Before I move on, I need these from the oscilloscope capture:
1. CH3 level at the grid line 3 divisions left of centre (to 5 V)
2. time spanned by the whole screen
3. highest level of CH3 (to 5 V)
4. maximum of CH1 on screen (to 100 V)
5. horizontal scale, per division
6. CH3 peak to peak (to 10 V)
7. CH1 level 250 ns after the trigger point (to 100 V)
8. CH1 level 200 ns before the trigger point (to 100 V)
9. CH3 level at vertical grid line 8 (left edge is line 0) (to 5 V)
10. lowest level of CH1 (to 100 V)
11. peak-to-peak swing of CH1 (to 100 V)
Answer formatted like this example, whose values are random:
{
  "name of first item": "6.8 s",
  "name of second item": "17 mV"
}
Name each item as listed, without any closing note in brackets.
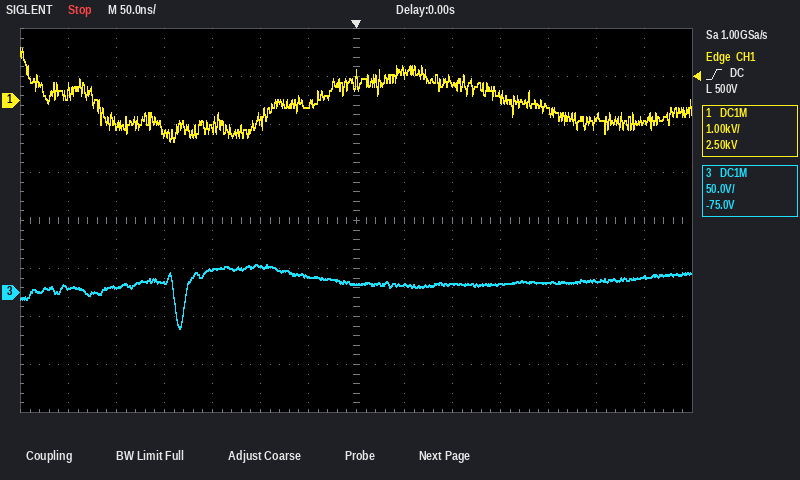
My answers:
{
  "CH3 level at the grid line 3 divisions left of centre": "25 V",
  "time spanned by the whole screen": "700 ns",
  "highest level of CH3": "30 V",
  "maximum of CH1 on screen": "1.1 kV",
  "horizontal scale, per division": "50 ns",
  "CH3 peak to peak": "70 V",
  "CH1 level 250 ns after the trigger point": "-400 V",
  "CH1 level 200 ns before the trigger point": "-700 V",
  "CH3 level at vertical grid line 8 (left edge is line 0)": "10 V",
  "lowest level of CH1": "-900 V",
  "peak-to-peak swing of CH1": "2.0 kV"
}
